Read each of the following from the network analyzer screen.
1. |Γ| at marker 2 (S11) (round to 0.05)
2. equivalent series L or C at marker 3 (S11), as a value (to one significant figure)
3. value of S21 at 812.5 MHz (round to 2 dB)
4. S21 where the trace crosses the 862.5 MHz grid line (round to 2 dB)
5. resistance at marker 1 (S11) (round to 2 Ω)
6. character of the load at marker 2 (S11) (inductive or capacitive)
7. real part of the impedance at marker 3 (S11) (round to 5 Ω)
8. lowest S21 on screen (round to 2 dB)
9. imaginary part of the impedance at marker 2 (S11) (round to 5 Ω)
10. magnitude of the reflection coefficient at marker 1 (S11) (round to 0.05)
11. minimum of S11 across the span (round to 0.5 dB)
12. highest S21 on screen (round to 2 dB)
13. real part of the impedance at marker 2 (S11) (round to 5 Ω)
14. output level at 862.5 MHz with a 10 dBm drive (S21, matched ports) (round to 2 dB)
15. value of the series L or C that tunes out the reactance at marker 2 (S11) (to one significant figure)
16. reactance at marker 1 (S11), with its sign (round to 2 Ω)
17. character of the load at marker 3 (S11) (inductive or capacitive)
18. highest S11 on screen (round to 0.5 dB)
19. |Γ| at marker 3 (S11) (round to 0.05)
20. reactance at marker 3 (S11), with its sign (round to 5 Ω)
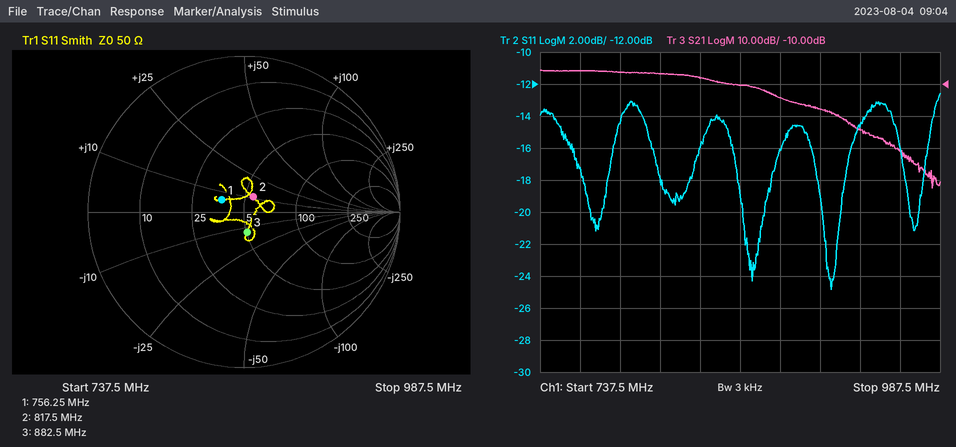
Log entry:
0.10
10 pF
-6 dB
-10 dB
38 Ω
inductive
50 Ω
-42 dB
+10 Ω
0.15
-25.0 dB
-6 dB
55 Ω
0 dBm
20 pF
+6 Ω
capacitive
-12.5 dB
0.15
-15 Ω
